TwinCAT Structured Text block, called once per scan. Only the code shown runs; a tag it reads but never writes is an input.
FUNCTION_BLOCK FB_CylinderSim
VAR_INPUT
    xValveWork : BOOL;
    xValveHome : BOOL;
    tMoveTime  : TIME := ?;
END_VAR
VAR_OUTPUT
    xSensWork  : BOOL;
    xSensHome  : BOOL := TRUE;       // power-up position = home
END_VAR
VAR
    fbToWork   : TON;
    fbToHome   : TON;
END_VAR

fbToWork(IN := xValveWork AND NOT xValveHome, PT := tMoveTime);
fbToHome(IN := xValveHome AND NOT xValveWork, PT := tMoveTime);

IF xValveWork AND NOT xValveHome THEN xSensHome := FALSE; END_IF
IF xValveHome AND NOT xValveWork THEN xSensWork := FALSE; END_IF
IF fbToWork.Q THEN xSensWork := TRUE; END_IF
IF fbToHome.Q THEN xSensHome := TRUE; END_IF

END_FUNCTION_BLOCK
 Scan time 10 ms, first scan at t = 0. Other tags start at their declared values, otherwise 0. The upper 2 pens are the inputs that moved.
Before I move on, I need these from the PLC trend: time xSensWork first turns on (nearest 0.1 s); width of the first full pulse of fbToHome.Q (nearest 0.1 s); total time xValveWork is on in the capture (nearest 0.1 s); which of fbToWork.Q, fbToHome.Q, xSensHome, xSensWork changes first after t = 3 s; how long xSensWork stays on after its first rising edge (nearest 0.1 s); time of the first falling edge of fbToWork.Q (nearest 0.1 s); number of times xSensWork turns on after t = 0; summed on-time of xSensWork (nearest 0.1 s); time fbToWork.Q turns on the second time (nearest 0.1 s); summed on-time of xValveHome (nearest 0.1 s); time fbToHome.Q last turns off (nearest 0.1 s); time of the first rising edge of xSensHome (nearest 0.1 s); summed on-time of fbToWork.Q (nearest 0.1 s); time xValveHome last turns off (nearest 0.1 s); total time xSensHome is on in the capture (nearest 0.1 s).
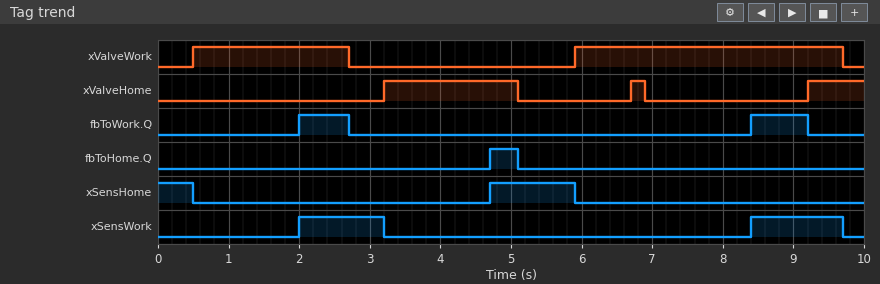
2.0 s
0.4 s
6.0 s
xSensWork
1.2 s
2.7 s
2
2.5 s
8.4 s
2.9 s
5.1 s
4.7 s
1.5 s
6.9 s
1.7 s
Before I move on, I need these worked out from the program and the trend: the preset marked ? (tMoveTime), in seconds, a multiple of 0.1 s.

1.5 s
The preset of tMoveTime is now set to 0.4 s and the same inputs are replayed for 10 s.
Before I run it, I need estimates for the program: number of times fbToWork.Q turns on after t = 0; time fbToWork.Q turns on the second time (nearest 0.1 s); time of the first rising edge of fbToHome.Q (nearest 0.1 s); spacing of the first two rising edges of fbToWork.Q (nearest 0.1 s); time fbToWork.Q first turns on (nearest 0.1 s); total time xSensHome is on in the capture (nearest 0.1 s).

3
6.3 s
3.6 s
5.4 s
0.9 s
2.8 s
